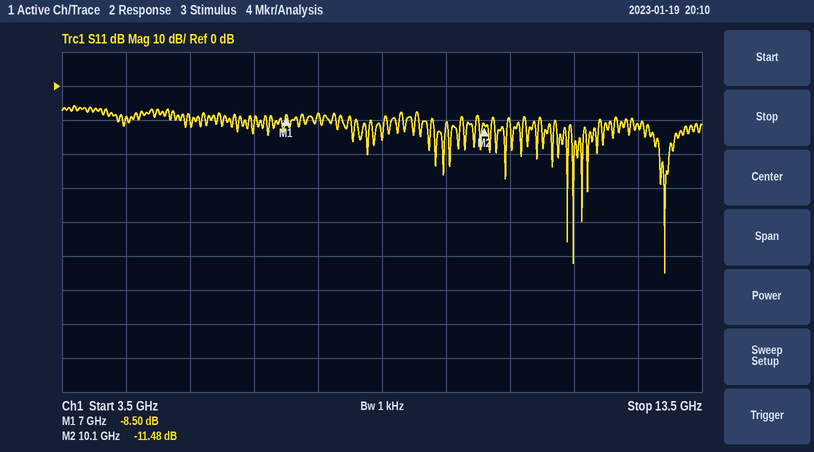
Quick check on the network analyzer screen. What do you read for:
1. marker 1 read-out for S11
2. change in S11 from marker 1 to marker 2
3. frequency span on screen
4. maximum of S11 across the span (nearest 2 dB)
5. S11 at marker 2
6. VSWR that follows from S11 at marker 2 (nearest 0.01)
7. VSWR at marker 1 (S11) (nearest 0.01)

-8.50 dB
-2.98 dB
10 GHz
-6 dB
-11.48 dB
1.73
2.20
